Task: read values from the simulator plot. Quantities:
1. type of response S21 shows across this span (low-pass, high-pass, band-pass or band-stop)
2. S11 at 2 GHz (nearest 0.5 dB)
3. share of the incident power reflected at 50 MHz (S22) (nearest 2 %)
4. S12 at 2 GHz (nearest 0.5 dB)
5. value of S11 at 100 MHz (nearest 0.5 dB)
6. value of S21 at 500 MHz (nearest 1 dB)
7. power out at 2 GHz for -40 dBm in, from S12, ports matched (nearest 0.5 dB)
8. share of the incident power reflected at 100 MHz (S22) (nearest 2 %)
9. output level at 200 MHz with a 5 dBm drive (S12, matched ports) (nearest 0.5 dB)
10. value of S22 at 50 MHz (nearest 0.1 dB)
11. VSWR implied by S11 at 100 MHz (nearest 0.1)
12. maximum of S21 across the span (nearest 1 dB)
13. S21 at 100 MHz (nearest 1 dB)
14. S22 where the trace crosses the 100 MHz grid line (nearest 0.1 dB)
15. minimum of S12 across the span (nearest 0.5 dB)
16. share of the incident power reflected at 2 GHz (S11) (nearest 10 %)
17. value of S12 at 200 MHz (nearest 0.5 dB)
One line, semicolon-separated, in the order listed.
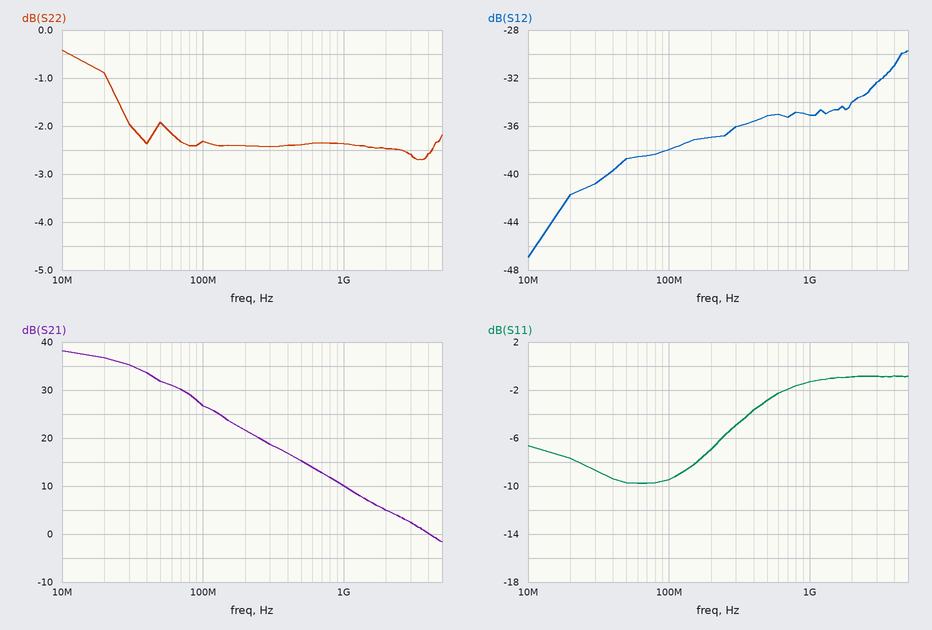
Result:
low-pass; -1.0 dB; 64 %; -34.0 dB; -9.5 dB; 15 dB; -74.0 dBm; 58 %; -32.0 dBm; -1.9 dB; 2.0; 38 dB; 27 dB; -2.3 dB; -47.0 dB; 80 %; -37.0 dB
